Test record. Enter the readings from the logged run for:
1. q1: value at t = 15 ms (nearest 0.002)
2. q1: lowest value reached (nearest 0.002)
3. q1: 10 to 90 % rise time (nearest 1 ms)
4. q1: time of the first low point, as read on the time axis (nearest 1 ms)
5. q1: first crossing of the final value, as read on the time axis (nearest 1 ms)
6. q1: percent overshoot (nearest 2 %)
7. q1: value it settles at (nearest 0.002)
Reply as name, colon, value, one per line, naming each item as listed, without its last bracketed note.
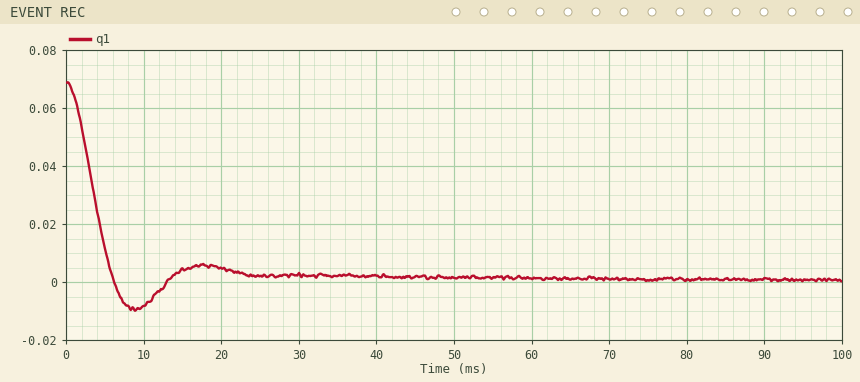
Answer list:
q1: value at t = 15 ms: 0.004
q1: lowest value reached: -0.010
q1: 10 to 90 % rise time: 4 ms
q1: time of the first low point, as read on the time axis: 9 ms
q1: first crossing of the final value, as read on the time axis: 6 ms
q1: percent overshoot: 14 %
q1: value it settles at: 0.000
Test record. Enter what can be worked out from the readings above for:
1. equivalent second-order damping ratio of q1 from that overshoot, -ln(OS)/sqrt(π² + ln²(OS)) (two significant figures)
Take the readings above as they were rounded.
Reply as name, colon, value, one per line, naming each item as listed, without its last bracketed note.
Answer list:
equivalent second-order damping ratio of q1 from that overshoot, -ln(OS)/sqrt(π² + ln²(OS)): 0.53
